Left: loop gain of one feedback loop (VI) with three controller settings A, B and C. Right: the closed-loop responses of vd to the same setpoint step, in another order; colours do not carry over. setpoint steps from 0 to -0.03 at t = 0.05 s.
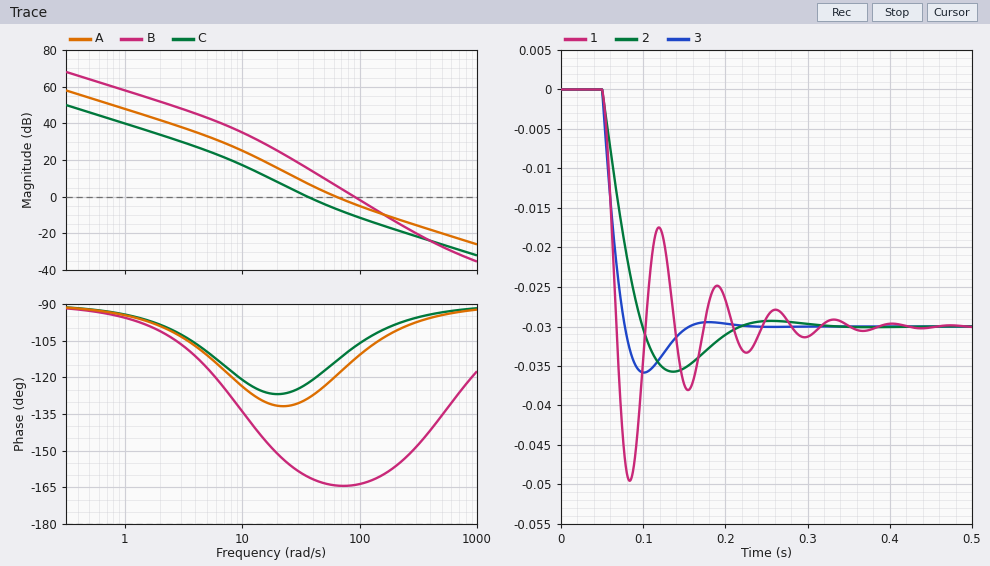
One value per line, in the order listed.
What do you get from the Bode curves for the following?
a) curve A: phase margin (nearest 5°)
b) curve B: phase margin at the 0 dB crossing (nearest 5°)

60°
15°
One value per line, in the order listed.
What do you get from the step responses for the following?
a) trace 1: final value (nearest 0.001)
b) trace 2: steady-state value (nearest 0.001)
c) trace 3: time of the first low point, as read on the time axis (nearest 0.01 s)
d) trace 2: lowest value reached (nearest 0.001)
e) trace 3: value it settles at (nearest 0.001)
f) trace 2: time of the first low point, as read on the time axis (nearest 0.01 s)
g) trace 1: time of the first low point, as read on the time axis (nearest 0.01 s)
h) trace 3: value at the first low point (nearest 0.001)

-0.030
-0.030
0.10 s
-0.036
-0.030
0.14 s
0.08 s
-0.036
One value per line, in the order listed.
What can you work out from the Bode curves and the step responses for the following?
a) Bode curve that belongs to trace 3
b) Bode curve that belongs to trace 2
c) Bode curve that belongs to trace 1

A
C
B
